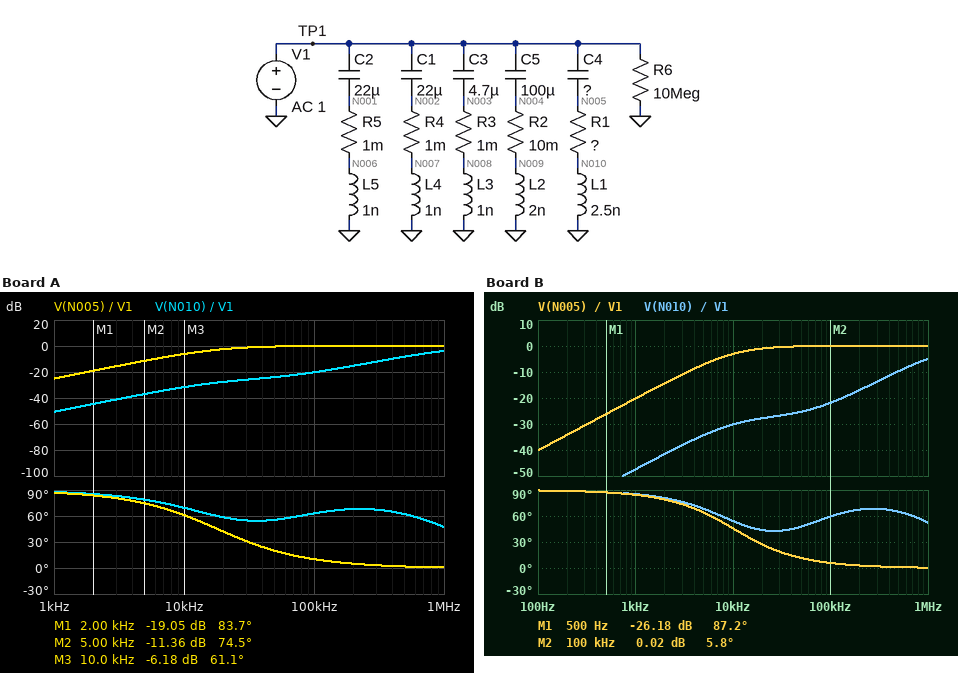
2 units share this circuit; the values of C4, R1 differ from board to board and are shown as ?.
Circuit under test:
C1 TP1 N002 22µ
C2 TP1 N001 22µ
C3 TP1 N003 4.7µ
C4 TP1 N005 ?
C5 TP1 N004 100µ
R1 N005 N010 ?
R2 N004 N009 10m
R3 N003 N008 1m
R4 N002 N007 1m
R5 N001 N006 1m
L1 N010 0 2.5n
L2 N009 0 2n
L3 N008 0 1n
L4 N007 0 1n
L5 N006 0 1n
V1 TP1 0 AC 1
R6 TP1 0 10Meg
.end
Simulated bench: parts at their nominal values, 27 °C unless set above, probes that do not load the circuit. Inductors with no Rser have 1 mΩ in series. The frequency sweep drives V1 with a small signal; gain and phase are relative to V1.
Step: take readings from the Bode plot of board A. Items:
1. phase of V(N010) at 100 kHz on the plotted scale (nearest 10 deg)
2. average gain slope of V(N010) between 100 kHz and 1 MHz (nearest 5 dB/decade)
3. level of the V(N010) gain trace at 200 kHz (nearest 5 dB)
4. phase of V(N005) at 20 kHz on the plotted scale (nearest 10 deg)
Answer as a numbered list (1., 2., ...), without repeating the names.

1. 60 deg
2. 15 dB/decade
3. -15 dB
4. 40 deg
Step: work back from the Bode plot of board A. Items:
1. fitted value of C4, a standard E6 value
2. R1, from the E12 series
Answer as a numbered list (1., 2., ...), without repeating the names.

1. 470 µF
2. 0.018 Ω
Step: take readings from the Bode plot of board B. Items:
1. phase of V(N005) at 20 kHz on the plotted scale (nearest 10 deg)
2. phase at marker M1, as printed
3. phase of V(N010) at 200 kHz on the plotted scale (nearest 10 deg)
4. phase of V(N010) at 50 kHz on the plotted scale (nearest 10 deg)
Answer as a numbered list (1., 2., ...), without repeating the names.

1. 30 deg
2. 87.2 deg
3. 70 deg
4. 50 deg
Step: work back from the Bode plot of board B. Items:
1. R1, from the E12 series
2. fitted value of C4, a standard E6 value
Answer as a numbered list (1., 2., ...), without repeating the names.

1. 0.022 Ω
2. 680 µF
